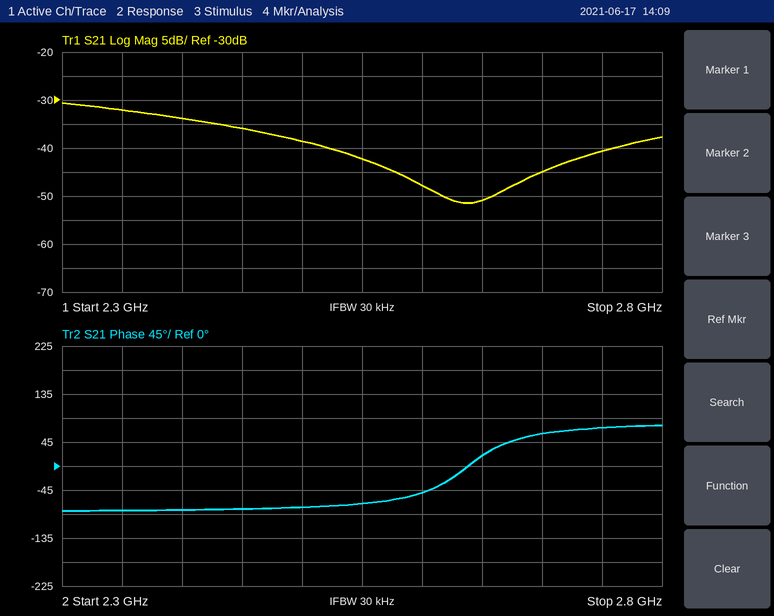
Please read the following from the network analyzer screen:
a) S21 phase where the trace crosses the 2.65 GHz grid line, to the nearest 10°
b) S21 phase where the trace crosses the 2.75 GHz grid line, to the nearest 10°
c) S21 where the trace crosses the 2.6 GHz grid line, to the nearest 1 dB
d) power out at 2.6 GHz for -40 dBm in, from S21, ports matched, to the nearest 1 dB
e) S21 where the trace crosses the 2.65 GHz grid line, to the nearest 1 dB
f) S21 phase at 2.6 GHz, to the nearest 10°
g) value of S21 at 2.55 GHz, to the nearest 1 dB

20°
70°
-48 dB
-88 dBm
-51 dB
-50°
-42 dB
